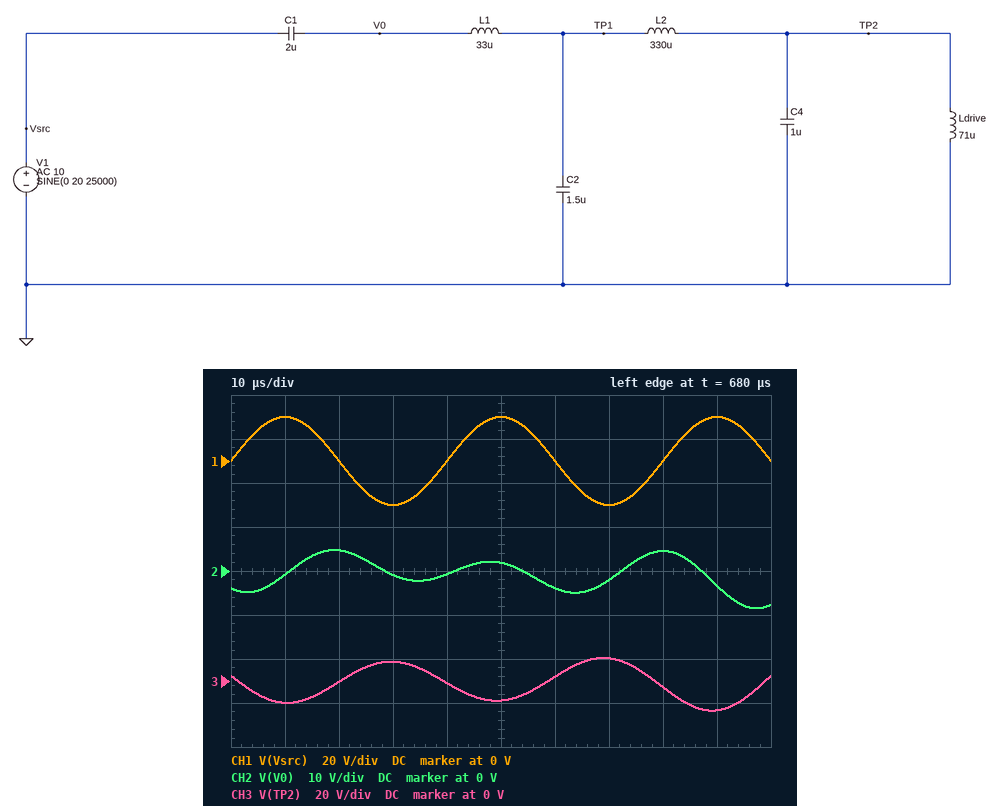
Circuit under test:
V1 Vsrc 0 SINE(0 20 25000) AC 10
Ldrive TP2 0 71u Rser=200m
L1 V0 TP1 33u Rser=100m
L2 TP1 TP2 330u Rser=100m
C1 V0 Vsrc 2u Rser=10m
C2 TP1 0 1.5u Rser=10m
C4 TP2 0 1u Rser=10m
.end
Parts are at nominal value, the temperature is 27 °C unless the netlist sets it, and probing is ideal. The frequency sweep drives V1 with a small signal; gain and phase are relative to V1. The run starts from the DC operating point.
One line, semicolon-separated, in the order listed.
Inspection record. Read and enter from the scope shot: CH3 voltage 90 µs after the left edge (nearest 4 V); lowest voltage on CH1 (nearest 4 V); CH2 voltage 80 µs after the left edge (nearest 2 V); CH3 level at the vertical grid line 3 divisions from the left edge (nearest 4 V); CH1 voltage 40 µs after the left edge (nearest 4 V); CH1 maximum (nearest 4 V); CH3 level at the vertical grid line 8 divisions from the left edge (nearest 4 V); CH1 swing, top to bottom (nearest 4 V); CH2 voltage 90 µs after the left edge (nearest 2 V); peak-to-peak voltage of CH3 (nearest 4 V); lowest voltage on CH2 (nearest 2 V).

-12 V; -20 V; 4 V; 8 V; 0 V; 20 V; -4 V; 40 V; -4 V; 24 V; -8 V
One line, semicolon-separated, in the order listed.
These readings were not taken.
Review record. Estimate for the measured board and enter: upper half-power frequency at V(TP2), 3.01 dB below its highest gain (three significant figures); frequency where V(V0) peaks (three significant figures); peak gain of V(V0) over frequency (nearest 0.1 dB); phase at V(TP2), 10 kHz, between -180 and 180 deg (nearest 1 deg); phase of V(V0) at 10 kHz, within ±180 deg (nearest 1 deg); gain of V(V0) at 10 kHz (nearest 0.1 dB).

21.0 kHz; 30.5 kHz; 26.6 dB; -3 deg; 0 deg; -3.6 dB
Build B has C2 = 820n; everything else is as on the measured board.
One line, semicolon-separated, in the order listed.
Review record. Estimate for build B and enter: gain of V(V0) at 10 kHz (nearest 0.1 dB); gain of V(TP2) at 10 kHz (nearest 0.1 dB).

-1.0 dB; -13.5 dB
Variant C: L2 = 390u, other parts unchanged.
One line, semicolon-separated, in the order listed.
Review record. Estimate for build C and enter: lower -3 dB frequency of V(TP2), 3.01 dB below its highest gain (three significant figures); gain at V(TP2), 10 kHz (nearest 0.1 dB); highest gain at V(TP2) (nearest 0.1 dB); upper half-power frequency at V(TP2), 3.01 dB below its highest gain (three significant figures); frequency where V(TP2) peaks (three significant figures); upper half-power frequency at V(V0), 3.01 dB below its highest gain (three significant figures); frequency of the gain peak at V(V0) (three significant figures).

20.3 kHz; -16.6 dB; 18.1 dB; 20.7 kHz; 20.5 kHz; 30.7 kHz; 30.4 kHz
